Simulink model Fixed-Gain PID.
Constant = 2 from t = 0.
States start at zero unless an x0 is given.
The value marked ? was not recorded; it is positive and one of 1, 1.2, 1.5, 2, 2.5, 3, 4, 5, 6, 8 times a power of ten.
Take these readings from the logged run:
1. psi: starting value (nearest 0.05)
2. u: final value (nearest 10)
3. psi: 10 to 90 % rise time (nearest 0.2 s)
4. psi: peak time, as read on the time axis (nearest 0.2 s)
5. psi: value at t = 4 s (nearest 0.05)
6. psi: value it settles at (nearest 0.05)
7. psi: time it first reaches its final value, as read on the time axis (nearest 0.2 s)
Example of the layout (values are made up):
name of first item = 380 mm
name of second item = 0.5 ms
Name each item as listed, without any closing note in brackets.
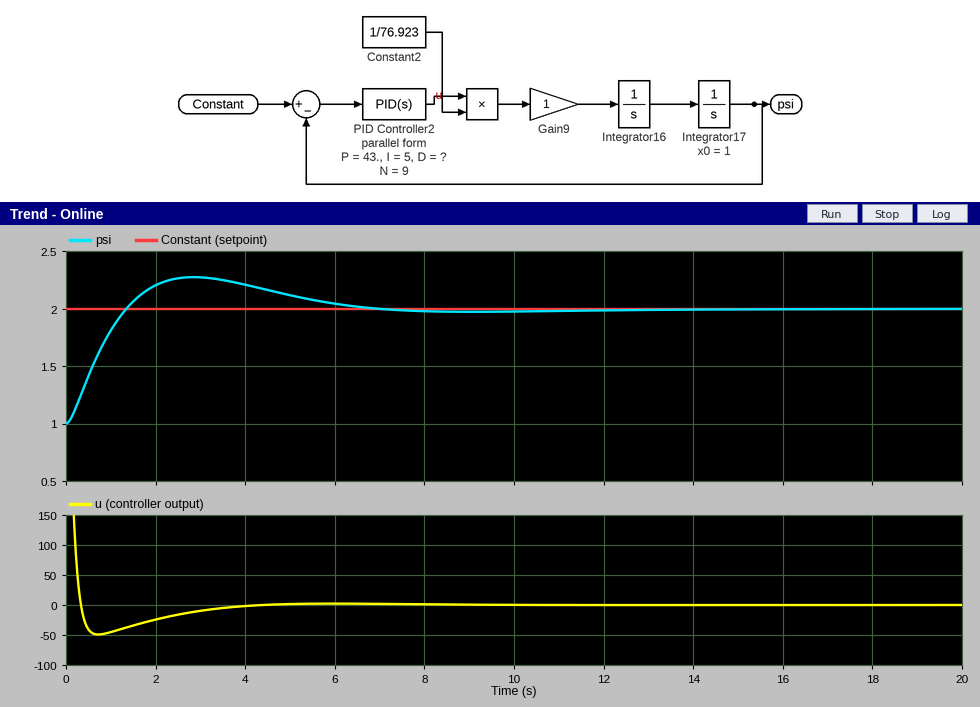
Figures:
psi: starting value = 1.00
u: final value = 0
psi: 10 to 90 % rise time = 1.0 s
psi: peak time, as read on the time axis = 2.8 s
psi: value at t = 4 s = 2.20
psi: value it settles at = 2.00
psi: time it first reaches its final value, as read on the time axis = 1.4 s
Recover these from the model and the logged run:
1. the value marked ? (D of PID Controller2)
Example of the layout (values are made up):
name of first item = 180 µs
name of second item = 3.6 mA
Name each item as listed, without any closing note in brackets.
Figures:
the value marked ? = 80
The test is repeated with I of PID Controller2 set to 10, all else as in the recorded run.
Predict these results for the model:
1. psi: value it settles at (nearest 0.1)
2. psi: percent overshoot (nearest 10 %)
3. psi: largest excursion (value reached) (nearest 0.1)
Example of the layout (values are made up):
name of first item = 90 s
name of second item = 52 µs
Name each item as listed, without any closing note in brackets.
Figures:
psi: value it settles at = 2.0
psi: percent overshoot = 30 %
psi: largest excursion (value reached) = 2.3
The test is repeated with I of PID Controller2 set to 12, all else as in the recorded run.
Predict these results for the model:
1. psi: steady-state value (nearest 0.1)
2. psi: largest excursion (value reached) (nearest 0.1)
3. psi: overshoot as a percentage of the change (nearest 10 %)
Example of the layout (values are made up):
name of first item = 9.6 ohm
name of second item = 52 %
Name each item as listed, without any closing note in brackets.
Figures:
psi: steady-state value = 2.0
psi: largest excursion (value reached) = 2.3
psi: overshoot as a percentage of the change = 30 %
